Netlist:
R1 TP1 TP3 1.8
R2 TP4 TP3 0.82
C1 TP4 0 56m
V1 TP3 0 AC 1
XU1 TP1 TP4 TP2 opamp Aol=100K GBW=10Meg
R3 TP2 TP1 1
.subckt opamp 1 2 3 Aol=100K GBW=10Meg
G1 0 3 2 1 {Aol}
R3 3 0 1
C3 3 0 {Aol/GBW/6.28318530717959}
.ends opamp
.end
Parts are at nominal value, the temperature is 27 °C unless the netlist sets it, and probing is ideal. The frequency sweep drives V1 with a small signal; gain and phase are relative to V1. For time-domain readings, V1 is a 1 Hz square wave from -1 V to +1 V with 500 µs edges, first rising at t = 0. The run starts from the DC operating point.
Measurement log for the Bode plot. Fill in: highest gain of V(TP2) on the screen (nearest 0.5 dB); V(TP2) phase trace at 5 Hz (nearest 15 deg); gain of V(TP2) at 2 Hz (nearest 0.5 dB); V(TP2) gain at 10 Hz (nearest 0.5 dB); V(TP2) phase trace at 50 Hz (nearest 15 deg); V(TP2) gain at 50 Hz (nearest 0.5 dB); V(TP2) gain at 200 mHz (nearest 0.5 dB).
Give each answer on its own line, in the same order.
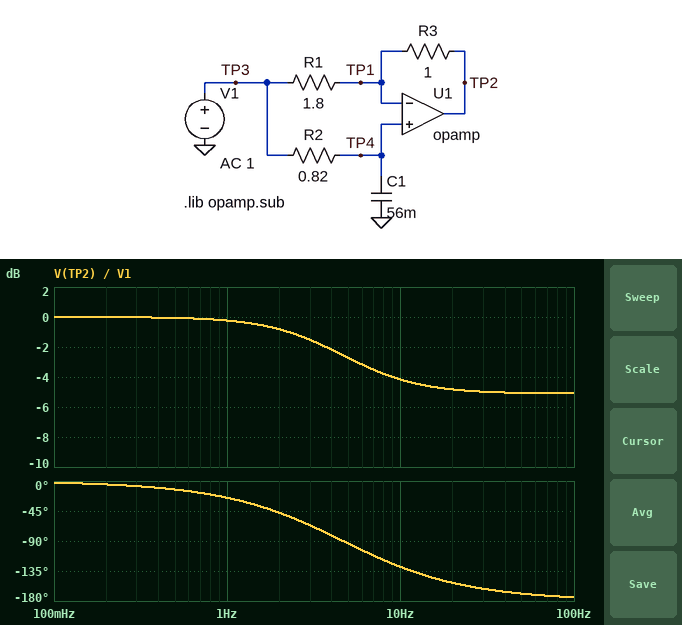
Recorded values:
0 dB
-90 deg
-1.0 dB
-4.0 dB
-165 deg
-5.0 dB
0 dB
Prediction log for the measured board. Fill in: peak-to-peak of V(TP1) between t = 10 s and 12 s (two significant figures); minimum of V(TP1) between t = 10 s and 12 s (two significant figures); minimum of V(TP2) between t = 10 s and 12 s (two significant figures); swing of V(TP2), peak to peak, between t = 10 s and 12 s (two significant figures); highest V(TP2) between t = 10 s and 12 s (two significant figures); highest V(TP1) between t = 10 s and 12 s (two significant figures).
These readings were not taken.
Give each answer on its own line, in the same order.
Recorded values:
2.0 V
-1.0 V
-2.1 V
4.2 V
2.1 V
1.0 V
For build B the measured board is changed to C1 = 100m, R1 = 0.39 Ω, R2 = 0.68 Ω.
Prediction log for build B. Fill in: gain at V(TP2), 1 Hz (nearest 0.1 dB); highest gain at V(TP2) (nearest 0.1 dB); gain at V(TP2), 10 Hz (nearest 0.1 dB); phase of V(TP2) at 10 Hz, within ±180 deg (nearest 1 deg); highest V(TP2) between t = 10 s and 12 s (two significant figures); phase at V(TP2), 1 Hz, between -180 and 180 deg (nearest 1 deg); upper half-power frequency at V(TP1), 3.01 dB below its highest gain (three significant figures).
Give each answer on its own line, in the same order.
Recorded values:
2.7 dB
8.2 dB
8.0 dB
-162 deg
6.1 V
-71 deg
2.34 Hz
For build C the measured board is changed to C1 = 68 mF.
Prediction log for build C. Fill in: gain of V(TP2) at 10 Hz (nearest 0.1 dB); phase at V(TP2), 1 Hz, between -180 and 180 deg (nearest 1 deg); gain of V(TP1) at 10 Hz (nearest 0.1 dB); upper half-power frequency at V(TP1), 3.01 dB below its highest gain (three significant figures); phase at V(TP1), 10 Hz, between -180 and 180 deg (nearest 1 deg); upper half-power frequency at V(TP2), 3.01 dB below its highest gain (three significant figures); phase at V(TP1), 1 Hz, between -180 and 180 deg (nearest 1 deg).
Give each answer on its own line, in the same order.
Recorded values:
-4.4 dB
-30 deg
-11.2 dB
2.85 Hz
-74 deg
4.61 Hz
-19 deg
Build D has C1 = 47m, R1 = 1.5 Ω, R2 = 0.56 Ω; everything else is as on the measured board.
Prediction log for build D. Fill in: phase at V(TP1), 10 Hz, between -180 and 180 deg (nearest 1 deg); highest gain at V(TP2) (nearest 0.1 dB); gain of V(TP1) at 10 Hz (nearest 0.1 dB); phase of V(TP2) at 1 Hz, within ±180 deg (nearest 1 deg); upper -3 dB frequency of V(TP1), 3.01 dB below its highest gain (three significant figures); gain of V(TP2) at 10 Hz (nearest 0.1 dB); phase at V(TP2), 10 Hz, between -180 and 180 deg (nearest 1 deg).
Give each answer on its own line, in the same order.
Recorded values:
-59 deg
0 dB
-5.7 dB
-16 deg
6.05 Hz
-2.3 dB
-107 deg
